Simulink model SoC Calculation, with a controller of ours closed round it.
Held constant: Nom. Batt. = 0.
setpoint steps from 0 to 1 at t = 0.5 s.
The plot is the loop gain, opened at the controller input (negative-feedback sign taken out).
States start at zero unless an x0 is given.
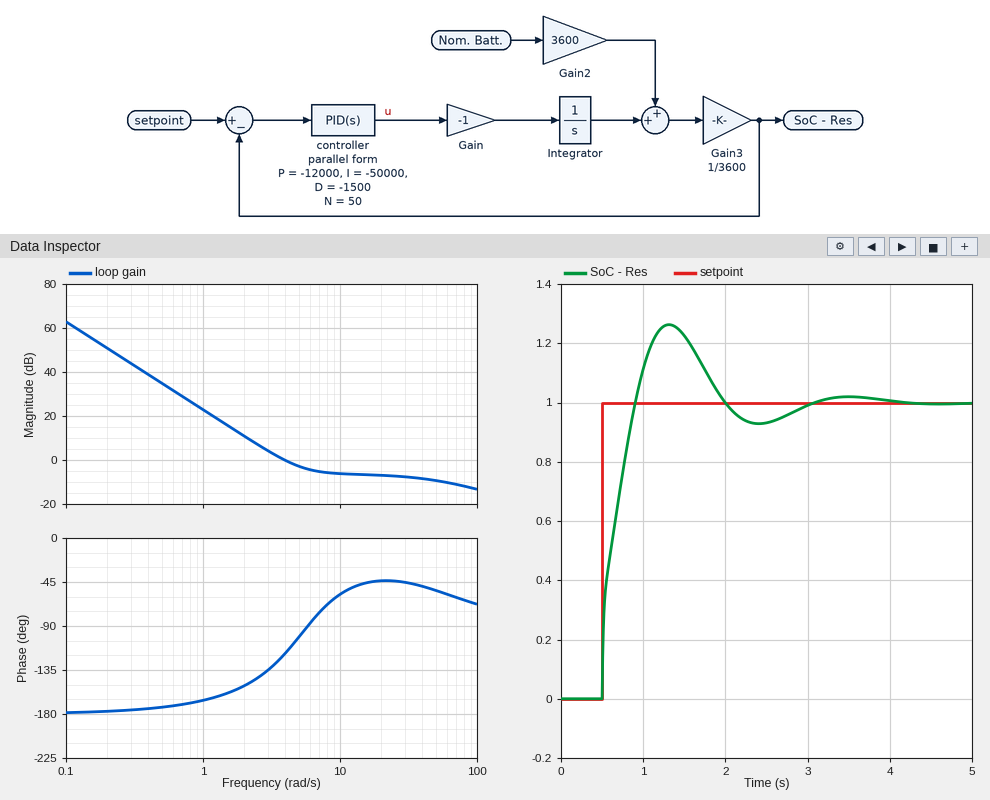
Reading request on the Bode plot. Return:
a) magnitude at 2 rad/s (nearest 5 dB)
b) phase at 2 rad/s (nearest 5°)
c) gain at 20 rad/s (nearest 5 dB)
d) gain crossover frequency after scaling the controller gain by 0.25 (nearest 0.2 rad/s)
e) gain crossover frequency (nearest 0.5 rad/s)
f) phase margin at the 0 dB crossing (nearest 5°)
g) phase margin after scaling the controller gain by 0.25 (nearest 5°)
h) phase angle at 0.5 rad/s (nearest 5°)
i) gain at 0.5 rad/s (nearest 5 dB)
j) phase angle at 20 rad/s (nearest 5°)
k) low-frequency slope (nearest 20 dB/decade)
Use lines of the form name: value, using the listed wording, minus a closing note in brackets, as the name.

magnitude at 2 rad/s: 10 dB
phase at 2 rad/s: -150°
gain at 20 rad/s: -5 dB
gain crossover frequency after scaling the controller gain by 0.25: 1.8 rad/s
gain crossover frequency: 4.0 rad/s
phase margin at the 0 dB crossing: 60°
phase margin after scaling the controller gain by 0.25: 25°
phase angle at 0.5 rad/s: -175°
gain at 0.5 rad/s: 35 dB
phase angle at 20 rad/s: -45°
low-frequency slope: -40 dB/decade
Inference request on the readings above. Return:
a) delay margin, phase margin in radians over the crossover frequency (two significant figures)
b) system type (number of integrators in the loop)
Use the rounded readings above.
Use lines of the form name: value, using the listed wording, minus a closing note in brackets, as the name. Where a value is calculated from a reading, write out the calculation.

delay margin, phase margin in radians over the crossover frequency: 60 × π / 180 / 4 = 0.26 s
system type: 2
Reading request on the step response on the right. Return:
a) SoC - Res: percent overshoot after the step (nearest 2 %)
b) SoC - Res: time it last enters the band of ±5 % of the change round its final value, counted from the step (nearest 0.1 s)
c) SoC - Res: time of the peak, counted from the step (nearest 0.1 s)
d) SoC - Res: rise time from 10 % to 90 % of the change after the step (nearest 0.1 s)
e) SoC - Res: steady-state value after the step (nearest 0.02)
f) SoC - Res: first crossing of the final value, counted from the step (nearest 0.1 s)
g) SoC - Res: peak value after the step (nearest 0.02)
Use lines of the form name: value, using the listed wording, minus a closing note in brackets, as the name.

SoC - Res: percent overshoot after the step: 26 %
SoC - Res: time it last enters the band of ±5 % of the change round its final value, counted from the step: 2.2 s
SoC - Res: time of the peak, counted from the step: 0.8 s
SoC - Res: rise time from 10 % to 90 % of the change after the step: 0.3 s
SoC - Res: steady-state value after the step: 1.00
SoC - Res: first crossing of the final value, counted from the step: 0.4 s
SoC - Res: peak value after the step: 1.26
